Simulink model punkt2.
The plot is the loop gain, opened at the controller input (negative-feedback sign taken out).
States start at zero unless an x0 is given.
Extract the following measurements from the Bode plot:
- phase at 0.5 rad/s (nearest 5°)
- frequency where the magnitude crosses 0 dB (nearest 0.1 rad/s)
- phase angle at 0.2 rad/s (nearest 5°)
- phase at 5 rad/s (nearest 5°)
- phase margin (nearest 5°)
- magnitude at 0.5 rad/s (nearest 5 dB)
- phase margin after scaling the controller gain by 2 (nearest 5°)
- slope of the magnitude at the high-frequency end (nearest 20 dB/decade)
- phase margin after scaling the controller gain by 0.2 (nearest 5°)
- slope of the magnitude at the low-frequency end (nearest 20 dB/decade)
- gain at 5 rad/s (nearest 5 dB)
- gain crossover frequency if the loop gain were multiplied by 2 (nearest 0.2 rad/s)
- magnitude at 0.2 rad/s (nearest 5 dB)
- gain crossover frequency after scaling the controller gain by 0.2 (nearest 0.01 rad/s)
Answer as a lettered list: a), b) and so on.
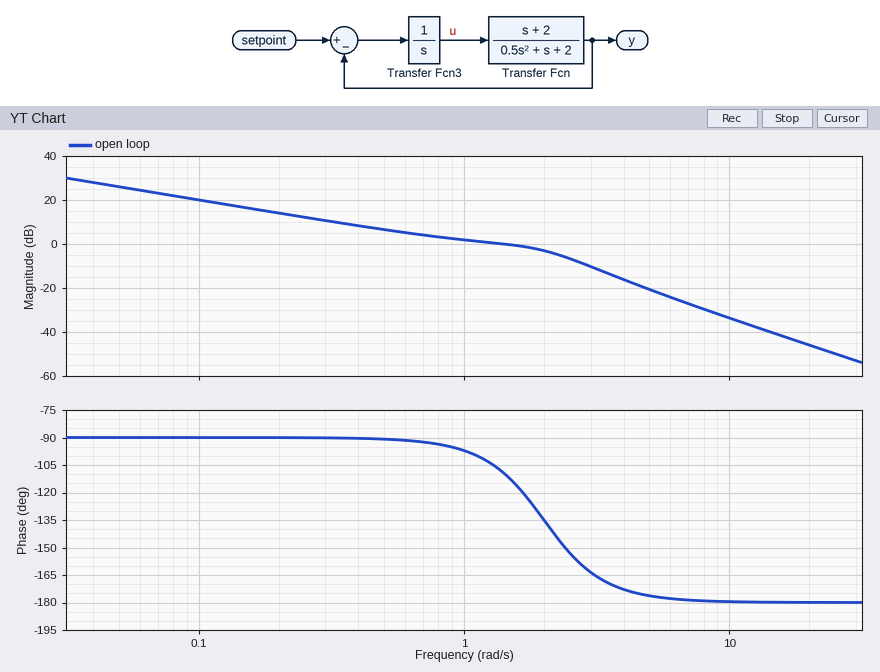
a) -90°
b) 1.4 rad/s
c) -90°
d) -175°
e) 70°
f) 5 dB
g) 30°
h) -40 dB/decade
i) 90°
j) -20 dB/decade
k) -20 dB
l) 2.4 rad/s
m) 15 dB
n) 0.20 rad/s
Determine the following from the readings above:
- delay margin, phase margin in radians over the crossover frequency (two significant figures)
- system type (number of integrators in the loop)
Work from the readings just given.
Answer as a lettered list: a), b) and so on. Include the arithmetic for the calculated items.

a) 70 × π / 180 / 1.4 = 0.87 s
b) 1
